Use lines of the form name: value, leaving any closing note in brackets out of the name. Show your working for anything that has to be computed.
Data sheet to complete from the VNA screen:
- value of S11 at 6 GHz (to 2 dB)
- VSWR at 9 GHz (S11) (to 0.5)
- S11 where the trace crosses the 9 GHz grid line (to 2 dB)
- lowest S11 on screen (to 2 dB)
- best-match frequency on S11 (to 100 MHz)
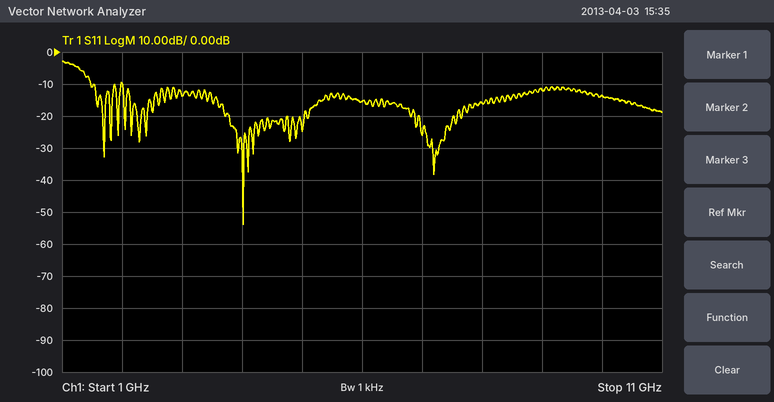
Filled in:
value of S11 at 6 GHz: -16 dB
VSWR at 9 GHz (S11): |Γ| = 10^(-12/20) = 0.2512; VSWR = (1 + 0.2512)/(1 − 0.2512) ≈ 1.67, so 1.5 to the nearest 0.5
S11 where the trace crosses the 9 GHz grid line: -12 dB
lowest S11 on screen: -54 dB
best-match frequency on S11: 4.0 GHz
